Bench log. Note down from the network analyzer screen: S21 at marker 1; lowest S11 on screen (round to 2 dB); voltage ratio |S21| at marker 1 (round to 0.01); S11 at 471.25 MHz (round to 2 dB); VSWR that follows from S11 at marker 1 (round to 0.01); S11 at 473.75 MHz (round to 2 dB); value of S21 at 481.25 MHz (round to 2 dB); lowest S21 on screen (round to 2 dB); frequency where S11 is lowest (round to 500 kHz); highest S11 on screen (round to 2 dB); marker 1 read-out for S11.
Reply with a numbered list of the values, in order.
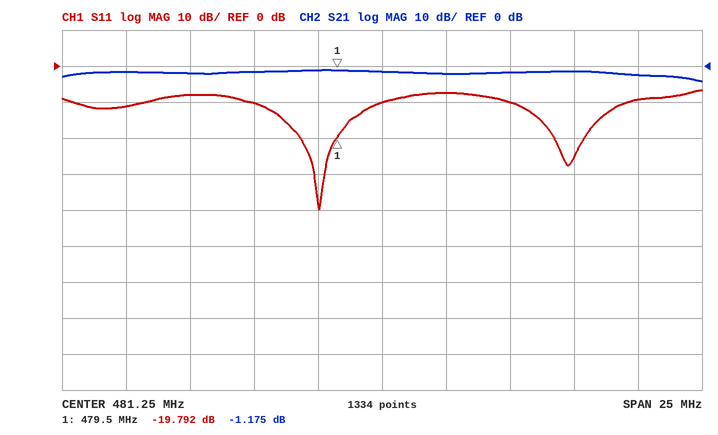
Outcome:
1. -1.175 dB
2. -40 dB
3. 0.87
4. -12 dB
5. 1.23
6. -8 dB
7. -2 dB
8. -4 dB
9. 479.0 MHz
10. -6 dB
11. -19.792 dB
